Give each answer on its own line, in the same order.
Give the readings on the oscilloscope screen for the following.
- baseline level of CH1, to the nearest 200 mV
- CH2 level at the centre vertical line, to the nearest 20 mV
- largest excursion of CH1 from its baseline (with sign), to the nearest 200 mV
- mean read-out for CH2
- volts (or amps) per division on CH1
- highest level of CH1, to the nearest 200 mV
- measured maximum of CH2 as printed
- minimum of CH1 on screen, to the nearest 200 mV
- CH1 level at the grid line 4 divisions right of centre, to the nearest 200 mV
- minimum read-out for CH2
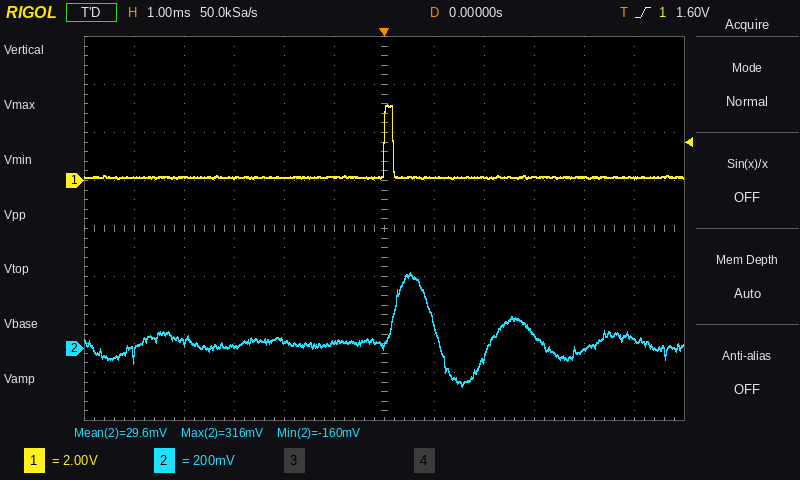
200 mV
20 mV
+3.0 V
29.6 mV
2 V
3.2 V
316 mV
0.0 V
200 mV
-160 mV
